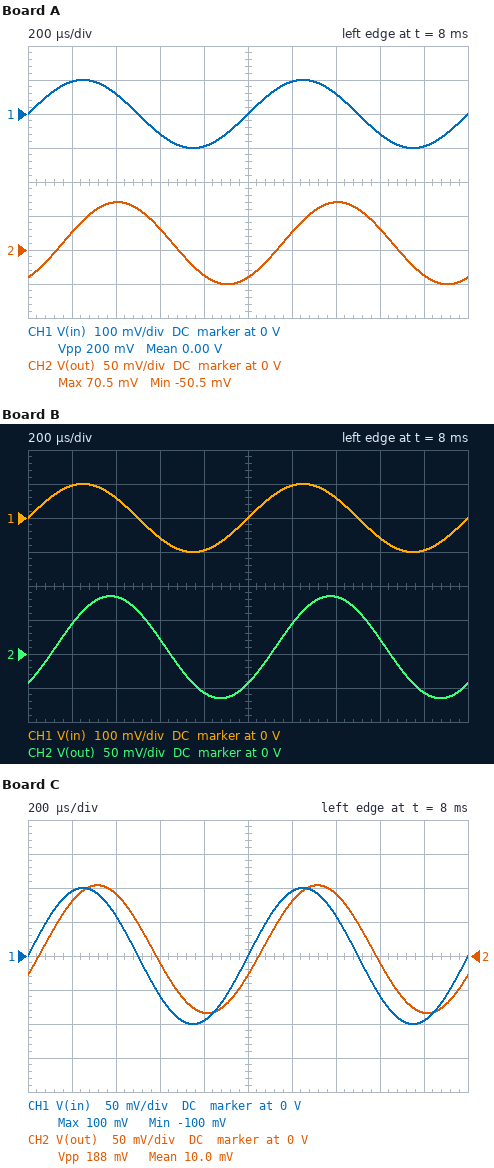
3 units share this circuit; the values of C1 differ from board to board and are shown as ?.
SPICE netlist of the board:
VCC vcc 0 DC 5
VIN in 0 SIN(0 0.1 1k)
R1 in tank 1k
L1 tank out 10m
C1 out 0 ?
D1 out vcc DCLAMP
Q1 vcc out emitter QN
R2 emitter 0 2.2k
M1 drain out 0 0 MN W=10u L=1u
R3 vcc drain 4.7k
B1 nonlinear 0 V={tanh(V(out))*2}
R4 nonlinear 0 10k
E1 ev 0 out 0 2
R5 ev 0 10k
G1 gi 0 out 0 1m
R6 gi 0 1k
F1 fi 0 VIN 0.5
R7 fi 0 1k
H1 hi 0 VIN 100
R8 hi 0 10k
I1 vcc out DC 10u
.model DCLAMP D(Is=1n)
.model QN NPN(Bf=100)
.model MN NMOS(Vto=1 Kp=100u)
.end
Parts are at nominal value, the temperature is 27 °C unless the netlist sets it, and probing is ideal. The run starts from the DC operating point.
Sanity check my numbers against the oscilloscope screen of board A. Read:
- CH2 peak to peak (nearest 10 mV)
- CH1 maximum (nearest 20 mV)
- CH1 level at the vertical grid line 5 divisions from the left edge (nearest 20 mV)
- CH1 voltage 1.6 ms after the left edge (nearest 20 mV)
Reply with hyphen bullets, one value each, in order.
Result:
- 120 mV
- 100 mV
- 0 V
- -60 mV
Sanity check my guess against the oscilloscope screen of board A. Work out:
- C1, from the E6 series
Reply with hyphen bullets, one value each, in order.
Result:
- 220 nF
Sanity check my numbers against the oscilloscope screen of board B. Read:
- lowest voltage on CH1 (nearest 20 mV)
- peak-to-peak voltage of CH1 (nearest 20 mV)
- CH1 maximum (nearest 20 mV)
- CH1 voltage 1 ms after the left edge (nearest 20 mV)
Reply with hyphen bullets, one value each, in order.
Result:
- -100 mV
- 200 mV
- 100 mV
- 0 V
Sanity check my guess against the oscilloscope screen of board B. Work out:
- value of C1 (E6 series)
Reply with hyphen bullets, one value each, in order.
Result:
- 150 nF
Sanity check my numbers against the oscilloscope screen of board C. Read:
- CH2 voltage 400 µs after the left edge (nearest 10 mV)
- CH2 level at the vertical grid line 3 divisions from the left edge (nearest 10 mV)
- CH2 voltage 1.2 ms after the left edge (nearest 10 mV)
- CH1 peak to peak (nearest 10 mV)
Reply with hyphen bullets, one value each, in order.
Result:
- 90 mV
- -10 mV
- 80 mV
- 200 mV
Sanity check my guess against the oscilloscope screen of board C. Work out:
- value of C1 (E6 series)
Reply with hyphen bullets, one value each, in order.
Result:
- 68 nF
